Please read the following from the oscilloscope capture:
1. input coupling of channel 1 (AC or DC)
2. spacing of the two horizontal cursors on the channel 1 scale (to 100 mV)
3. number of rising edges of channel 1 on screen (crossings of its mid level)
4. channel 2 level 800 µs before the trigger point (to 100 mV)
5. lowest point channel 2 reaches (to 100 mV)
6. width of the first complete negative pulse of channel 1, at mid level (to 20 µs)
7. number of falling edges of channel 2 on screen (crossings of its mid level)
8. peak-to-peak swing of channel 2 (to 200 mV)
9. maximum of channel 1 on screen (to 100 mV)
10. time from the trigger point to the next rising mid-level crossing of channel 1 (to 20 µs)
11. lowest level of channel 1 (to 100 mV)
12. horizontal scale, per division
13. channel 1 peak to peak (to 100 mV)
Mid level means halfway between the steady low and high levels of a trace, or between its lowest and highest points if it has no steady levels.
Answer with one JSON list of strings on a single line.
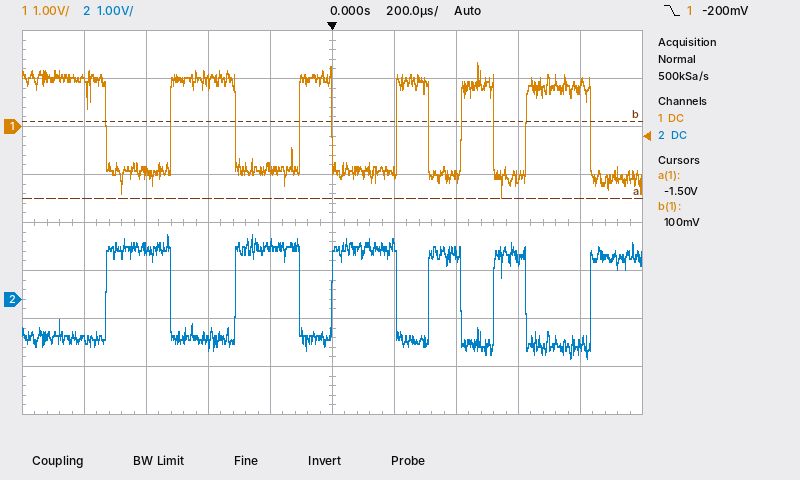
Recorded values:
["DC", "1.6 V", "5", "-800 mV", "-1.2 V", "200 µs", "5", "2.6 V", "1.3 V", "200 µs", "-1.5 V", "200 µs", "2.8 V"]
